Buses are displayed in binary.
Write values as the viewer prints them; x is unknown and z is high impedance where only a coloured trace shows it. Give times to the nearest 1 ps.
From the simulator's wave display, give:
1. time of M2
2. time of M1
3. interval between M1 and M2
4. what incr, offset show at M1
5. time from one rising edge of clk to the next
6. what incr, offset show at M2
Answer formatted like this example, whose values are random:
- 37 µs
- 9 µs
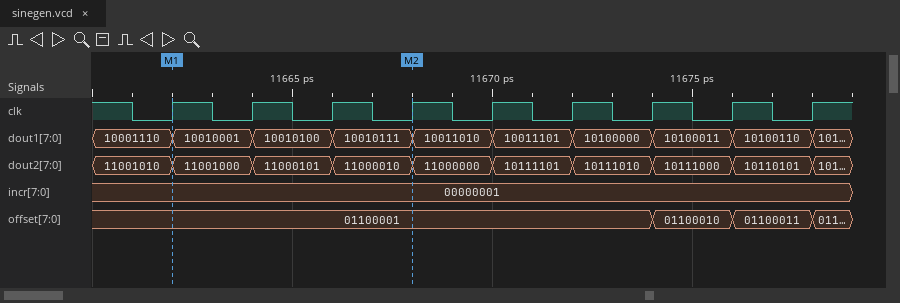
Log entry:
- 11668 ps
- 11662 ps
- 6 ps
- incr=00000001, offset=01100001
- 2 ps
- incr=00000001, offset=01100001
